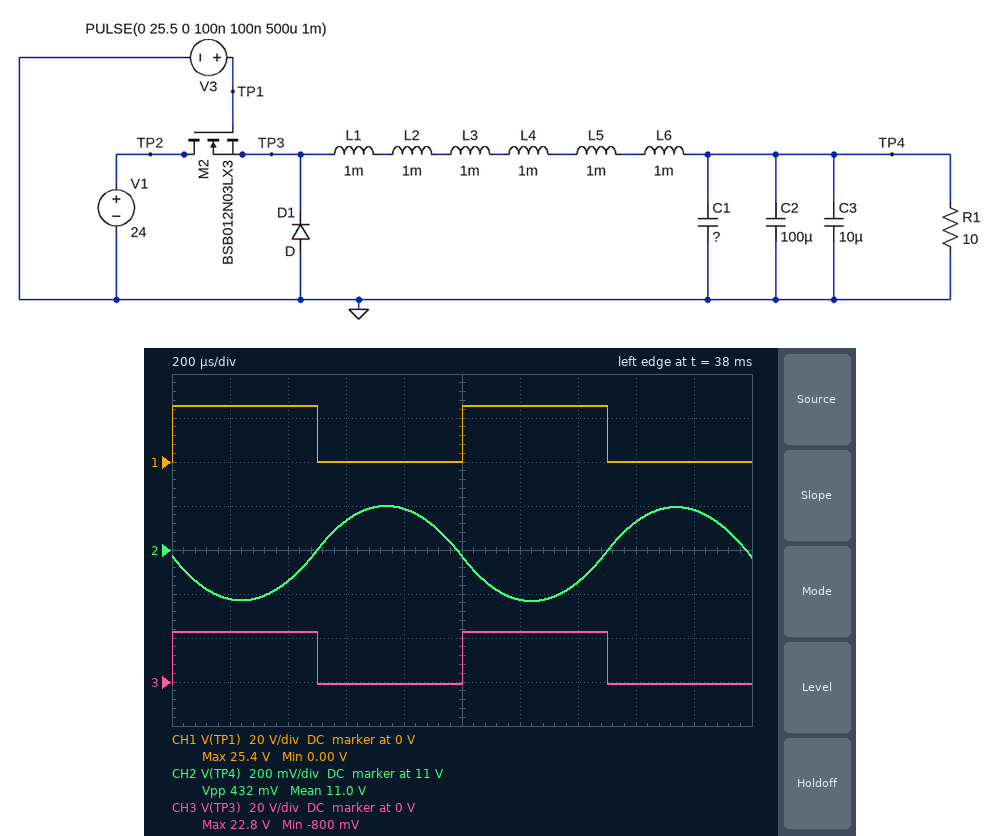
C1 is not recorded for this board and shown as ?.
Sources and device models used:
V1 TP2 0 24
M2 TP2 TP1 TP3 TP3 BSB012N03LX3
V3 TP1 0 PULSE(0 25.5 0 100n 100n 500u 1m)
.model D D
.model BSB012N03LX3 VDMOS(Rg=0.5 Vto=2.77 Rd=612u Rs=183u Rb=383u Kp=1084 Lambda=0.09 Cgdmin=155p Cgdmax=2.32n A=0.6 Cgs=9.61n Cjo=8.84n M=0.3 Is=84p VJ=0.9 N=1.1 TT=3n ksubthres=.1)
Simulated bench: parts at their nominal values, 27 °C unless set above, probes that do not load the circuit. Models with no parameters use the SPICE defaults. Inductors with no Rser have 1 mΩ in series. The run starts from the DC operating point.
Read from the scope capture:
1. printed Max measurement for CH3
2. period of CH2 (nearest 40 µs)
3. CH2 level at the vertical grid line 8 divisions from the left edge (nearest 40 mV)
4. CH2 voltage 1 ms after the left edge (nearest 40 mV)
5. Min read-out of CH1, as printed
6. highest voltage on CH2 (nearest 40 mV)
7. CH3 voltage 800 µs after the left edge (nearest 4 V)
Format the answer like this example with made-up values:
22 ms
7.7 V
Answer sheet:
22.8 V
1.00 ms
11.12 V
10.96 V
0.00 V
11.20 V
0 V
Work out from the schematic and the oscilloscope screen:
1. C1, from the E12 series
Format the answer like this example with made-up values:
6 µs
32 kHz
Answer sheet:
180 µF
